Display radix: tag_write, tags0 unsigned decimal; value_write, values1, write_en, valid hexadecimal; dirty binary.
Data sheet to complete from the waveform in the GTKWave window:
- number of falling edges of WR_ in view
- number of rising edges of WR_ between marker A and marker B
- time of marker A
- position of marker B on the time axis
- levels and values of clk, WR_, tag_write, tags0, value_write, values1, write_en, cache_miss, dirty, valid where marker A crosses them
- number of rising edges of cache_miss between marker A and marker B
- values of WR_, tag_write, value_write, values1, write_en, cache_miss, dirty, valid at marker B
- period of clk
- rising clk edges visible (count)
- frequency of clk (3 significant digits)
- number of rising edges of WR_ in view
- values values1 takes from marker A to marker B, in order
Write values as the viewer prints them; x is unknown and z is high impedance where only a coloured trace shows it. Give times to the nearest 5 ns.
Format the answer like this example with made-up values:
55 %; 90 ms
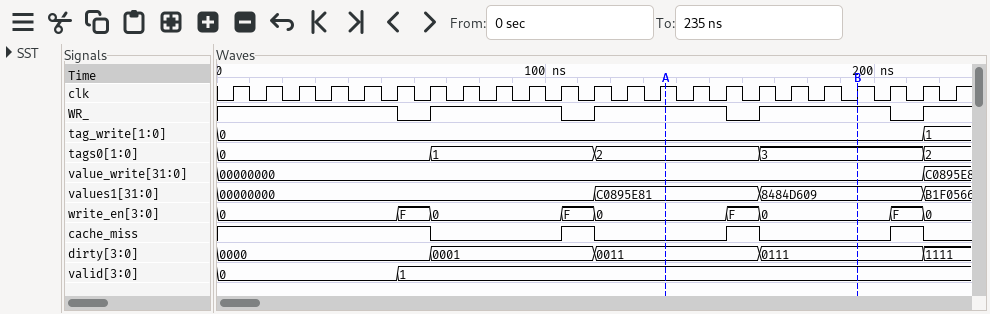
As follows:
4; 1; 135 ns; 195 ns; clk=1, WR_=1, tag_write=0, tags0=2, value_write=00000000, values1=C0895E81, write_en=0, cache_miss=0, dirty=0011, valid=1; 1; WR_=1, tag_write=0, value_write=00000000, values1=8484D609, write_en=0, cache_miss=0, dirty=0111, valid=1; 10 ns; 23; 100 MHz; 4; C0895E81, 8484D609
